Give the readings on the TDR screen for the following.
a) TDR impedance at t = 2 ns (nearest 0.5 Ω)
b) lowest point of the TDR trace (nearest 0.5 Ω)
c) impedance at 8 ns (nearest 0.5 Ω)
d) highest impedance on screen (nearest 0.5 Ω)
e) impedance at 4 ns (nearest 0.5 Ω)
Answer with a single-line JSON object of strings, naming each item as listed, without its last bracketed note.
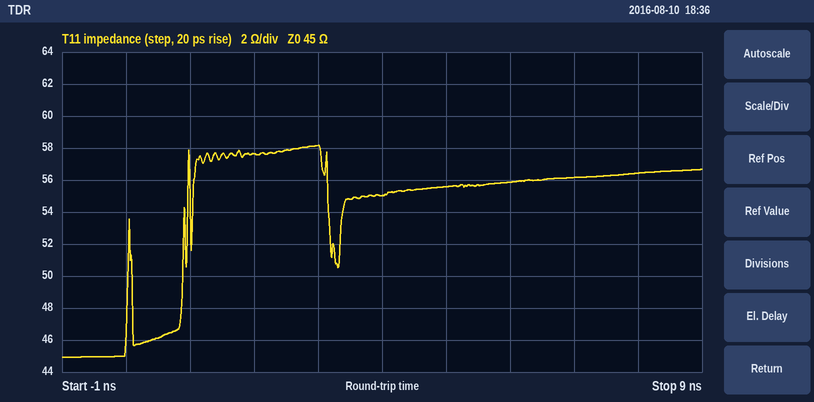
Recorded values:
{"TDR impedance at t = 2 ns": "57.5 Ω", "lowest point of the TDR trace": "45.0 Ω", "impedance at 8 ns": "56.5 Ω", "highest impedance on screen": "58.0 Ω", "impedance at 4 ns": "55.0 Ω"}
